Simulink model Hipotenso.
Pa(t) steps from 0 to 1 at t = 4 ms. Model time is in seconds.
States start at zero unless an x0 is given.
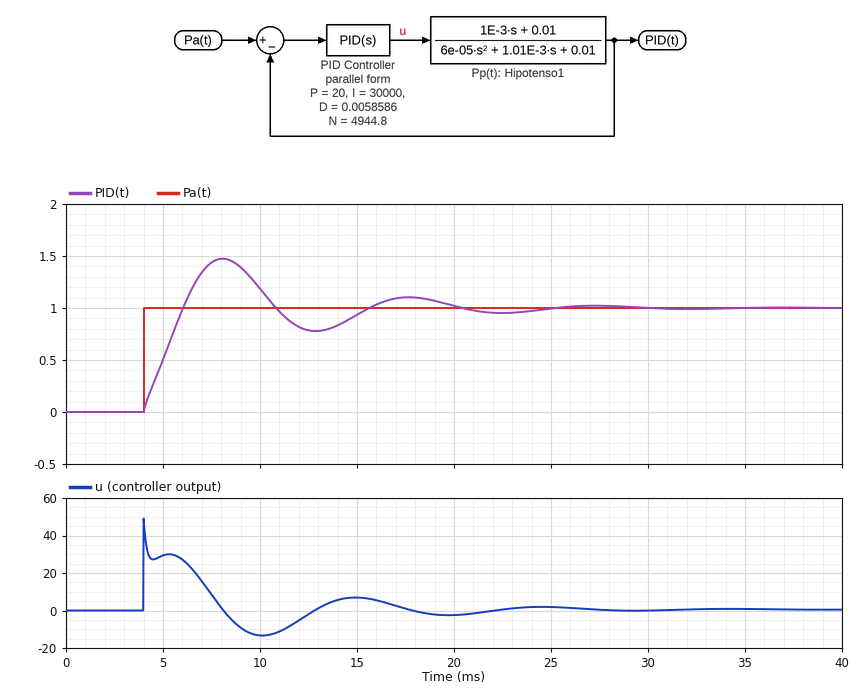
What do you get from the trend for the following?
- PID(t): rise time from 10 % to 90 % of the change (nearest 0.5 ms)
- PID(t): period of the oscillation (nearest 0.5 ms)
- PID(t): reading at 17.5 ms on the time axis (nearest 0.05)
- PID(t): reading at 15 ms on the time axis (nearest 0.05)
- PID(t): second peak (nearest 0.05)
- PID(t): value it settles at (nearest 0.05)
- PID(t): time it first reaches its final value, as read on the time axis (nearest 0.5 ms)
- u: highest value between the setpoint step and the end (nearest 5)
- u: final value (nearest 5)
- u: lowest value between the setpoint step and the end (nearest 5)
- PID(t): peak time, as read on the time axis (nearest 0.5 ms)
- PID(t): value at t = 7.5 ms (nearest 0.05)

1.5 ms
9.5 ms
1.10
0.95
1.10
1.00
6.0 ms
50
0
-15
8.0 ms
1.45
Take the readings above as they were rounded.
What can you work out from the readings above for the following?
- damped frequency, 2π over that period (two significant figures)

0.66 rad/ms
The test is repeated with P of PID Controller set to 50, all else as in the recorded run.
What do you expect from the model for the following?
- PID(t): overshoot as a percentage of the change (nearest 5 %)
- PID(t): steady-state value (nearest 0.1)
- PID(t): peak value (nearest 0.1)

25 %
1.0
1.2
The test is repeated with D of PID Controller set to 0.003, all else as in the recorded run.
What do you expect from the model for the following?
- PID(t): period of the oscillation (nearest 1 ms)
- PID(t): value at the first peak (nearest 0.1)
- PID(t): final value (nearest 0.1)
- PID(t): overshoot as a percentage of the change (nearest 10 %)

9 ms
1.5
1.0
50 %
